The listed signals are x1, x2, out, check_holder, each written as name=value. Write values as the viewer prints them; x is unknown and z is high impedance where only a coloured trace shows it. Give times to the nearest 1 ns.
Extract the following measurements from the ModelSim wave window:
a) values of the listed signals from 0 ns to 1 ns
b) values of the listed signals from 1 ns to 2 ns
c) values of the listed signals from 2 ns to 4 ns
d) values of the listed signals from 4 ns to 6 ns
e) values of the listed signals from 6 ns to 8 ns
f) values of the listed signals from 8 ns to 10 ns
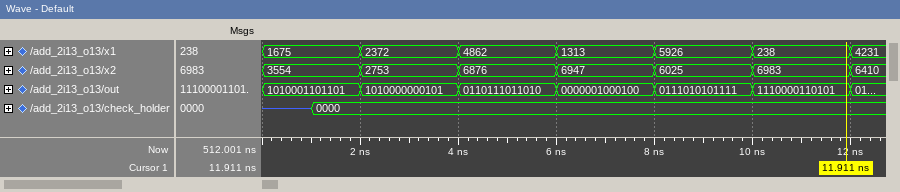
x1=1675, x2=3554, out=1010001101101, check_holder=z
x1=1675, x2=3554, out=1010001101101, check_holder=0000
x1=2372, x2=2753, out=1010000000101, check_holder=0000
x1=4862, x2=6876, out=0110111011010, check_holder=0000
x1=1313, x2=6947, out=0000001000100, check_holder=0000
x1=5926, x2=6025, out=0111010101111, check_holder=0000
